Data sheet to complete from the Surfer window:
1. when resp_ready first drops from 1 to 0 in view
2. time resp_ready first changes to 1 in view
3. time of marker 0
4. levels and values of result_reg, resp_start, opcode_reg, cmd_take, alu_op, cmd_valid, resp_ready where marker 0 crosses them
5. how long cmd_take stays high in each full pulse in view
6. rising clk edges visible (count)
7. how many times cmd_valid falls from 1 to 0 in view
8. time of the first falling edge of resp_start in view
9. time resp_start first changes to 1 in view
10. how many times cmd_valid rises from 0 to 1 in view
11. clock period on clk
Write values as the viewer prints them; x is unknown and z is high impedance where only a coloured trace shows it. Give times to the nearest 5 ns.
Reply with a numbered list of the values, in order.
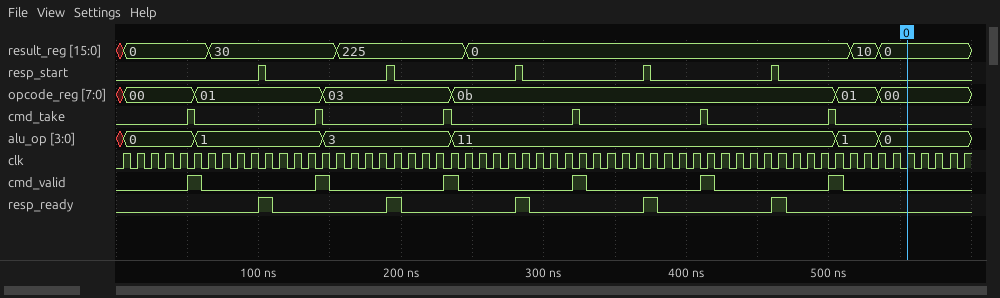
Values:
1. 110 ns
2. 100 ns
3. 555 ns
4. result_reg=0, resp_start=0, opcode_reg=00, cmd_take=0, alu_op=0, cmd_valid=0, resp_ready=0
5. 5 ns, 5 ns, 5 ns, 5 ns, 5 ns, 5 ns
6. 60
7. 6
8. 105 ns
9. 100 ns
10. 6
11. 10 ns
